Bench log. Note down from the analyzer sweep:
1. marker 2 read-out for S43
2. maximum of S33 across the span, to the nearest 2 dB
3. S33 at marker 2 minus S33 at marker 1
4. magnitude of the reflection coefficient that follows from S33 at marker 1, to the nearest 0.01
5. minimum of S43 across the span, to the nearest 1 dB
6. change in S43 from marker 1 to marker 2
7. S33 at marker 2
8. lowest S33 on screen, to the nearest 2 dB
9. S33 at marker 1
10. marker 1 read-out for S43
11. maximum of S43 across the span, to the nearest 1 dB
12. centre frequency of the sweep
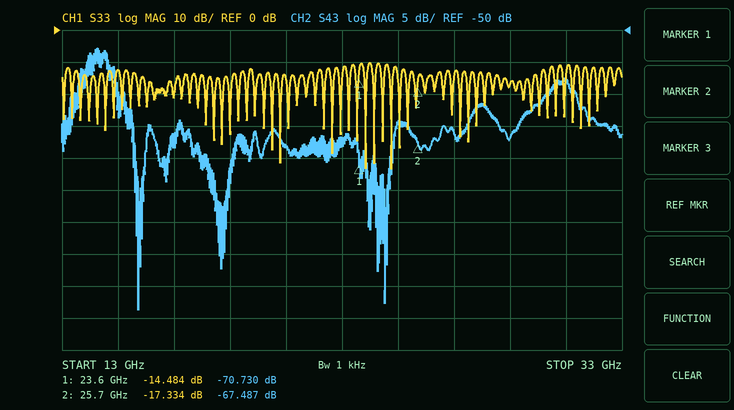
-67.487 dB
-10 dB
-2.850 dB
0.19
-94 dB
3.243 dB
-17.334 dB
-44 dB
-14.484 dB
-70.730 dB
-53 dB
23 GHz
